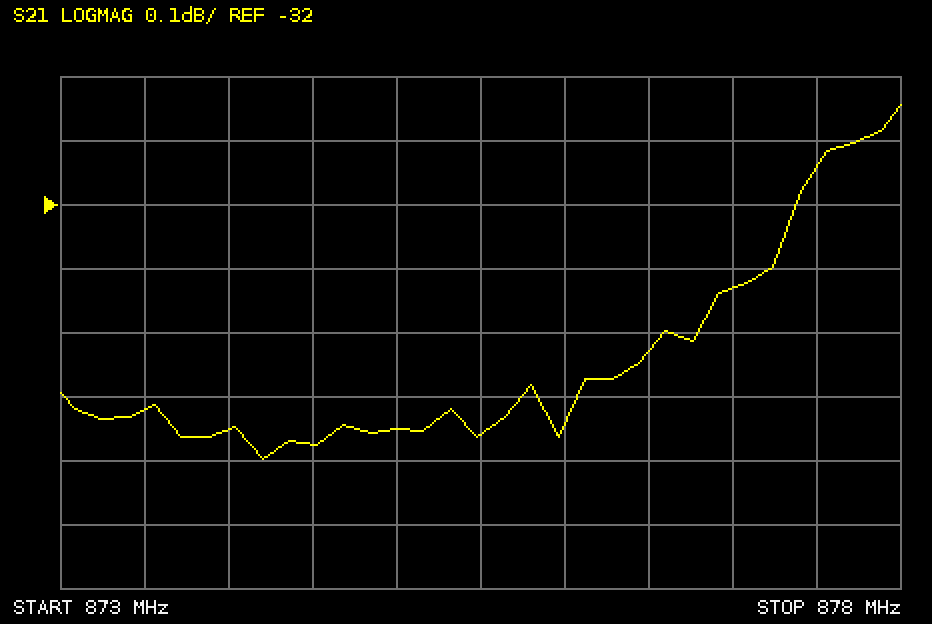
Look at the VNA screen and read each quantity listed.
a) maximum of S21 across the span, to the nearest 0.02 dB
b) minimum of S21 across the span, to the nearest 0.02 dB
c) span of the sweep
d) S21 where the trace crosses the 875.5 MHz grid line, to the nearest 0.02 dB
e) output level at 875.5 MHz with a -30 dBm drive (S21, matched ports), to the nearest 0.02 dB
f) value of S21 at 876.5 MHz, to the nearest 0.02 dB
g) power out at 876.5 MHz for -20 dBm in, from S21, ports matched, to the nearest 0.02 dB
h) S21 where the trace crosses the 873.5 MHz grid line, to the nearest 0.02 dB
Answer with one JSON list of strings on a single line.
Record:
["-31.84 dB", "-32.40 dB", "5 MHz", "-32.36 dB", "-62.36 dBm", "-32.22 dB", "-52.22 dBm", "-32.32 dB"]
